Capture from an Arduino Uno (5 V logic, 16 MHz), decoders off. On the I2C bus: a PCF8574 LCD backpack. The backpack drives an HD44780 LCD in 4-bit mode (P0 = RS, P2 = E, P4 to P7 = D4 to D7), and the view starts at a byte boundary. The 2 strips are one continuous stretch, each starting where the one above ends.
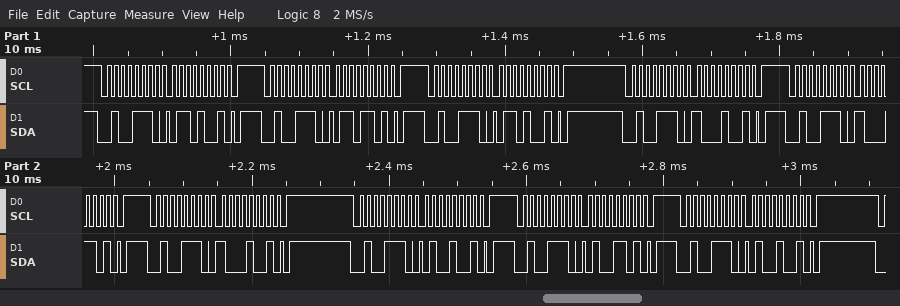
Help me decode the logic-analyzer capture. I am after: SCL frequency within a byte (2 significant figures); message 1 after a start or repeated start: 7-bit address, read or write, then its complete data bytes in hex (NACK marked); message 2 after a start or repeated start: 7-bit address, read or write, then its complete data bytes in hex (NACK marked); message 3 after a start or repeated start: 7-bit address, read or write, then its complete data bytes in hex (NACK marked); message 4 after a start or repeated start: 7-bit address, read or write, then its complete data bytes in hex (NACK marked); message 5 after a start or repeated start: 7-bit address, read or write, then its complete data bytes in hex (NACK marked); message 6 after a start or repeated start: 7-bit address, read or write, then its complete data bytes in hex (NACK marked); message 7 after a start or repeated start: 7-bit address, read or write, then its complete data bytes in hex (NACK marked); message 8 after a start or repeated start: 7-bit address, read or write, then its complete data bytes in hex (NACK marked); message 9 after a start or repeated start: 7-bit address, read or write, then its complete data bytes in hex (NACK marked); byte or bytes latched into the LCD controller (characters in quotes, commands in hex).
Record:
100 kHz
0x27 write: 69
0x27 write: 6D
0x27 write: 69
0x27 write: 89
0x27 write: 8D
0x27 write: 89
0x27 write: 49
0x27 write: 4D
0x27 write: 49
'h'
